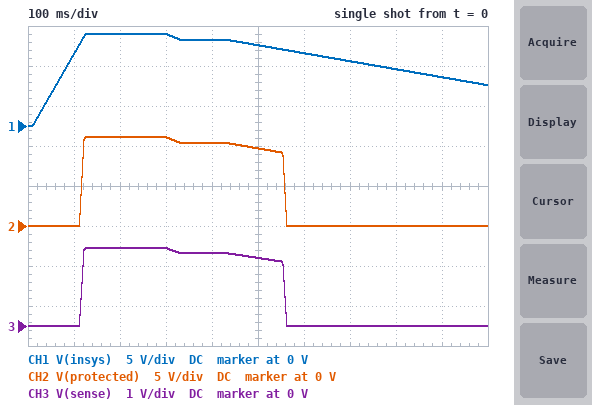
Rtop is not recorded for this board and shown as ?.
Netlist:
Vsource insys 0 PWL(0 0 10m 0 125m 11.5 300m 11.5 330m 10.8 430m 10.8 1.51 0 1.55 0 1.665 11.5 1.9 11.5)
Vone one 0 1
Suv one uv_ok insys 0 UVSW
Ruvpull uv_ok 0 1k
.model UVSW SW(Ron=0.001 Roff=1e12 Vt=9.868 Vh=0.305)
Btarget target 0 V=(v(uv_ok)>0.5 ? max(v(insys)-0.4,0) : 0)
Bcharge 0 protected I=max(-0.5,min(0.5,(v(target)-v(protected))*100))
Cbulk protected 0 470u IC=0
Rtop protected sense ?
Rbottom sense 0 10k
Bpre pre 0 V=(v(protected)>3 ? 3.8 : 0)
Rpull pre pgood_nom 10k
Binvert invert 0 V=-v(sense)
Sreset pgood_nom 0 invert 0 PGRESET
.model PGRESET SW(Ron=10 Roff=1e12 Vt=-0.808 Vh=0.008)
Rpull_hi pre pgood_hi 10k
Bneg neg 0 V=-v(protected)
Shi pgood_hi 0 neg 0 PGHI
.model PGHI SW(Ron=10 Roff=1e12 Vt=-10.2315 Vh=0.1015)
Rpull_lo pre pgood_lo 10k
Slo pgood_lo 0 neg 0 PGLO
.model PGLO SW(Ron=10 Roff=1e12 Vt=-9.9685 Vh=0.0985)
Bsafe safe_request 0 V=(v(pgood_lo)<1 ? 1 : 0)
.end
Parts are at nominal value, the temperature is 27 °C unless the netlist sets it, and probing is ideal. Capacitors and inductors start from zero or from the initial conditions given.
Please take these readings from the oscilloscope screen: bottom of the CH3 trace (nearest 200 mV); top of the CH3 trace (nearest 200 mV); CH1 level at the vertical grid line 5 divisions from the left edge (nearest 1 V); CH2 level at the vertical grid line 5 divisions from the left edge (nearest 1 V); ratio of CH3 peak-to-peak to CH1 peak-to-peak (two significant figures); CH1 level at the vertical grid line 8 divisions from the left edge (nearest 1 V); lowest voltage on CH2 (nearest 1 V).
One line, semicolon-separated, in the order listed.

0 V; 2.0 V; 10 V; 10 V; 0.17; 7 V; 0 V
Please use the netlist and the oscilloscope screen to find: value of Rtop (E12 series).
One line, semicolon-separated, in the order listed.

47 kΩ
